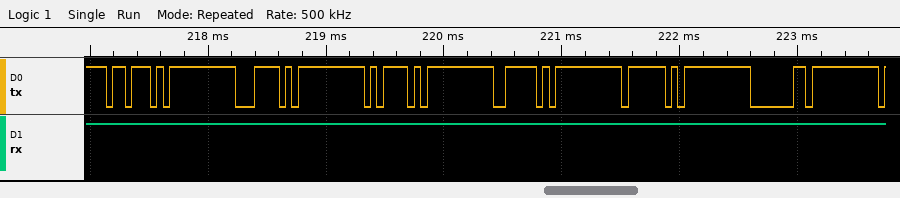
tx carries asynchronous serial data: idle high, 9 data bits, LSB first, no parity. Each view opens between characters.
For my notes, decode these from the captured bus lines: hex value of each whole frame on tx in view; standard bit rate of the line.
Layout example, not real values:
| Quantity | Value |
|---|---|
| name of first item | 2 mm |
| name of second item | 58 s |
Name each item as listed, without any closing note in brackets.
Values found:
| Quantity | Value |
|---|---|
| hex value of each whole frame on tx in view | BB, BC, BD, BE, BF, C0 |
| standard bit rate of the line | 19200 baud |
